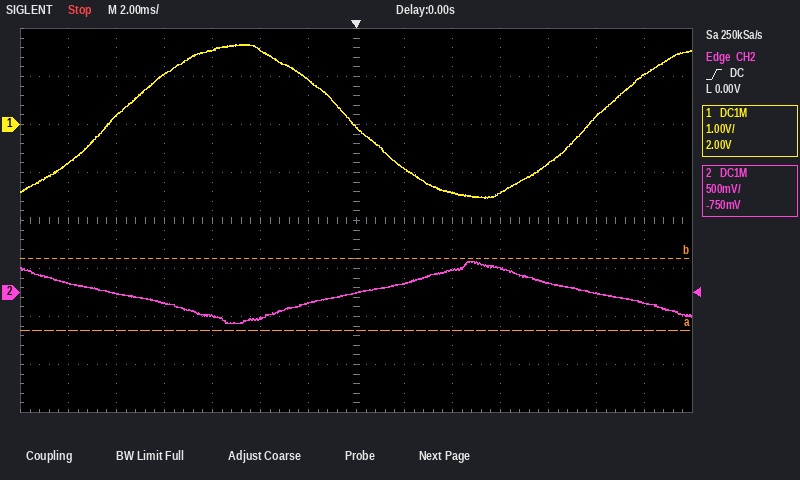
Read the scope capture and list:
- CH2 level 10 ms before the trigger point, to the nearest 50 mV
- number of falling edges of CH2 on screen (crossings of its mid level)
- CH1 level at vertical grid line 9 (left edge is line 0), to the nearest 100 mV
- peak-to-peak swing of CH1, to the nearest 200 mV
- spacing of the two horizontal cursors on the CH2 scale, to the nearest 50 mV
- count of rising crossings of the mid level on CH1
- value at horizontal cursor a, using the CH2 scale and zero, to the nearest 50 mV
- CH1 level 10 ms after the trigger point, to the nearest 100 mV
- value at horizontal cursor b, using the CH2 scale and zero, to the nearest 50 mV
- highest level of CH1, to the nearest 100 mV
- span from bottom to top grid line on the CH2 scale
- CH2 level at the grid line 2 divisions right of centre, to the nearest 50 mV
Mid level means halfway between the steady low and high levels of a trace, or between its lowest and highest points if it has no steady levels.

0 mV
2
-1.4 V
3.2 V
750 mV
2
-400 mV
200 mV
350 mV
1.7 V
4 V
250 mV
